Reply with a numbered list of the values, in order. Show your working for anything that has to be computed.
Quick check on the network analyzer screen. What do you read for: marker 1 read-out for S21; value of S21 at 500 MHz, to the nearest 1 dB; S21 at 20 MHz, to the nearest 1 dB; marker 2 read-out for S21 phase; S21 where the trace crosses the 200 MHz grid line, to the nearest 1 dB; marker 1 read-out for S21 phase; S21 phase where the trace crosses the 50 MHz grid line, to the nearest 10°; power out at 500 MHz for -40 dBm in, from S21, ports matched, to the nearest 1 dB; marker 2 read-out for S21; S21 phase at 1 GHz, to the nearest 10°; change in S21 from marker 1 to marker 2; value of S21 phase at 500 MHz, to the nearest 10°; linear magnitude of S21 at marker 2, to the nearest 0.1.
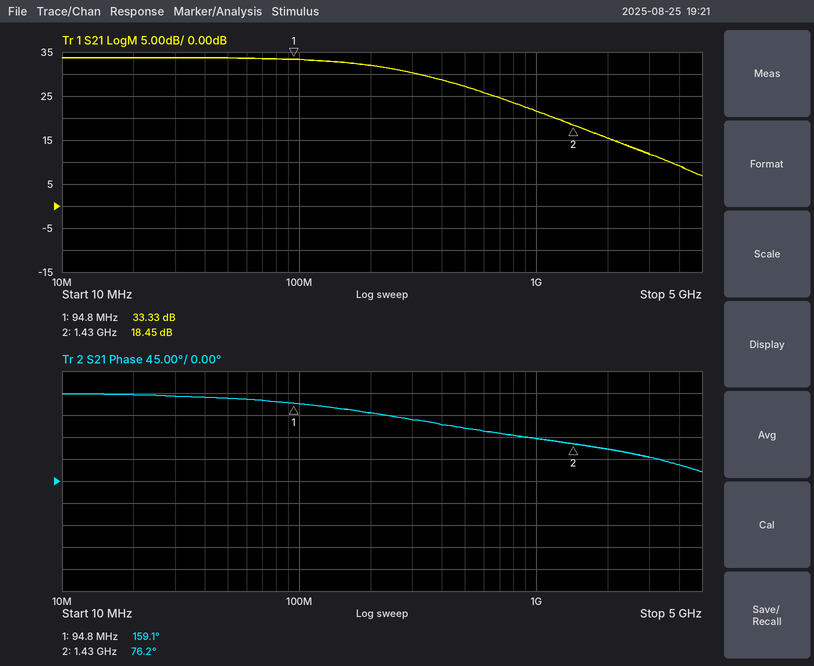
1. 33.33 dB
2. 27 dB
3. 34 dB
4. 76.2°
5. 32 dB
6. 159.1°
7. 170°
8. -40 dBm + (27 dB) = -13 dBm
9. 18.45 dB
10. 90°
11. 18.45 − (33.33) = -14.88 dB
12. 110°
13. 10^(18.45/20) ≈ 8.4
